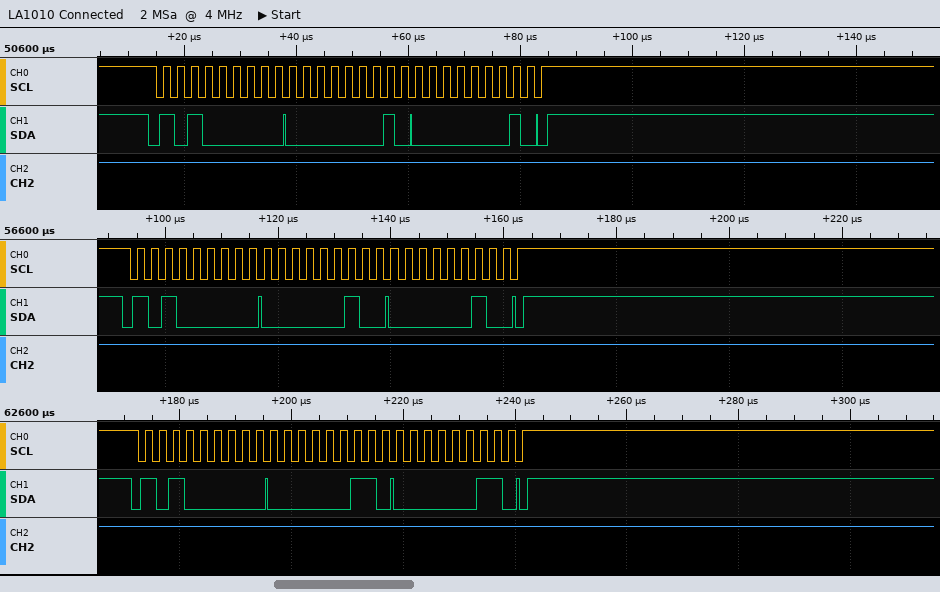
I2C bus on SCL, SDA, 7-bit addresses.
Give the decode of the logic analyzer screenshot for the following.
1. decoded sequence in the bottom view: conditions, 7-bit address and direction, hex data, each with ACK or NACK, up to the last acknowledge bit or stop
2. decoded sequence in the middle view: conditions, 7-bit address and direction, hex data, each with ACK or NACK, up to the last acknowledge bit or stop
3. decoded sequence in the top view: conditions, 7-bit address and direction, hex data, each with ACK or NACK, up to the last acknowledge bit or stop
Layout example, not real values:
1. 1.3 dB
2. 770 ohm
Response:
1. start, address 50 write ACK, 03 ACK, 03 ACK, stop
2. start, address 50 write ACK, 02 ACK, 02 ACK, stop
3. start, address 50 write ACK, 01 ACK, 01 ACK, stop
